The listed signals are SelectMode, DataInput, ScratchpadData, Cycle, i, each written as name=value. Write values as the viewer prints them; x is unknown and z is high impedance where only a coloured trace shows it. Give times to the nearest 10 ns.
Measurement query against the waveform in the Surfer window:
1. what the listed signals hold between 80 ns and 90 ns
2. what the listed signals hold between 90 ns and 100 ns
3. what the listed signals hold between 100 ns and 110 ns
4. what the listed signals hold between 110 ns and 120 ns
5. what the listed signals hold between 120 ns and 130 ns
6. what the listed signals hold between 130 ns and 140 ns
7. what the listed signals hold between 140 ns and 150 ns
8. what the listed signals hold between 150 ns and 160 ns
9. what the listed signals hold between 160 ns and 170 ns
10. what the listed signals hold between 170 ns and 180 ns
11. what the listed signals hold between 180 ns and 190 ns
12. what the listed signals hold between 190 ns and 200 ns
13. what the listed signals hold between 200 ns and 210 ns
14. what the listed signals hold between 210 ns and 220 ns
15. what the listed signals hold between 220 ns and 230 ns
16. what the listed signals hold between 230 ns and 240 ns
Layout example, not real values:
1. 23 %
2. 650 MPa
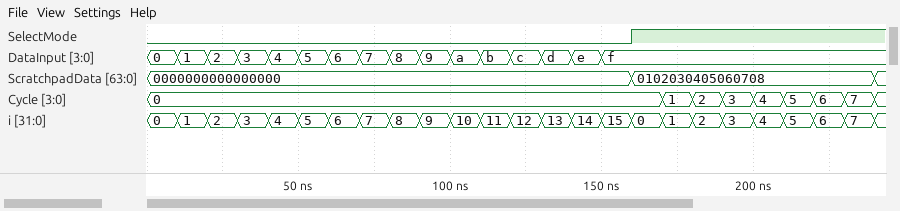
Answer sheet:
1. SelectMode=0, DataInput=8, ScratchpadData=0000000000000000, Cycle=0, i=8
2. SelectMode=0, DataInput=9, ScratchpadData=0000000000000000, Cycle=0, i=9
3. SelectMode=0, DataInput=a, ScratchpadData=0000000000000000, Cycle=0, i=10
4. SelectMode=0, DataInput=b, ScratchpadData=0000000000000000, Cycle=0, i=11
5. SelectMode=0, DataInput=c, ScratchpadData=0000000000000000, Cycle=0, i=12
6. SelectMode=0, DataInput=d, ScratchpadData=0000000000000000, Cycle=0, i=13
7. SelectMode=0, DataInput=e, ScratchpadData=0000000000000000, Cycle=0, i=14
8. SelectMode=0, DataInput=f, ScratchpadData=0000000000000000, Cycle=0, i=15
9. SelectMode=1, DataInput=f, ScratchpadData=0102030405060708, Cycle=0, i=0
10. SelectMode=1, DataInput=f, ScratchpadData=0102030405060708, Cycle=1, i=1
11. SelectMode=1, DataInput=f, ScratchpadData=0102030405060708, Cycle=2, i=2
12. SelectMode=1, DataInput=f, ScratchpadData=0102030405060708, Cycle=3, i=3
13. SelectMode=1, DataInput=f, ScratchpadData=0102030405060708, Cycle=4, i=4
14. SelectMode=1, DataInput=f, ScratchpadData=0102030405060708, Cycle=5, i=5
15. SelectMode=1, DataInput=f, ScratchpadData=0102030405060708, Cycle=6, i=6
16. SelectMode=1, DataInput=f, ScratchpadData=0102030405060708, Cycle=7, i=7
